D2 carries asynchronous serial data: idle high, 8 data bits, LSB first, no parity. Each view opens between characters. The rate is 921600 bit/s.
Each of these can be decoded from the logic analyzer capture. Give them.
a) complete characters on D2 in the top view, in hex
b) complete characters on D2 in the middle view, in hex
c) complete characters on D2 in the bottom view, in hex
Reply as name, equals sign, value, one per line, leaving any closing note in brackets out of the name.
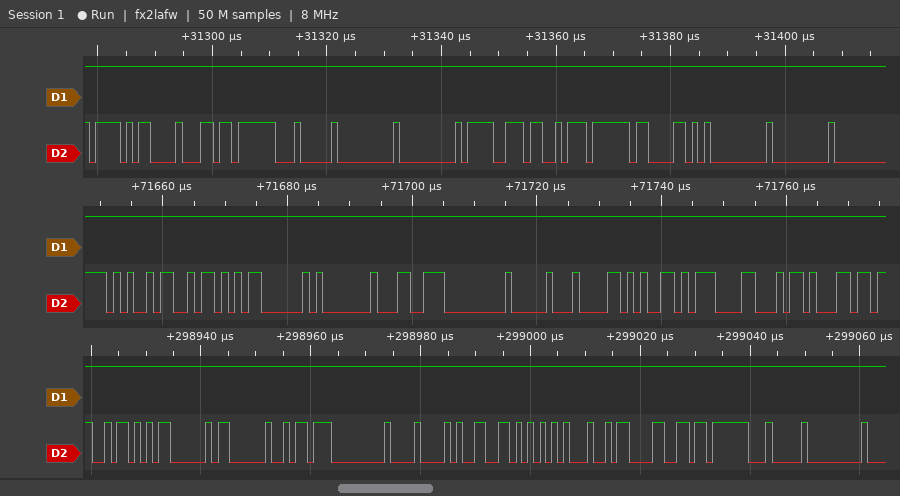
complete characters on D2 in the top view, in hex = AF, 88, FB, 04, 00, 00, CF, D3, BF, 58, 00, 00
complete characters on D2 in the middle view, in hex = A5, 5A, 03, 01, CC, 00, 10, 58, D6, 18, 8B
complete characters on D2 in the bottom view, in hex = 5A, 03, 03, DA, 00, 08, 99, 55, A4, 98, FB, 04, 00
